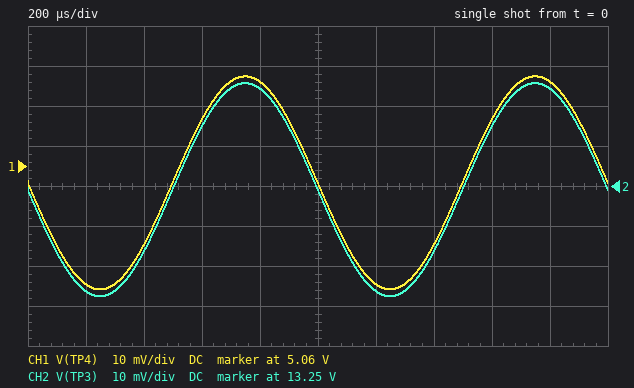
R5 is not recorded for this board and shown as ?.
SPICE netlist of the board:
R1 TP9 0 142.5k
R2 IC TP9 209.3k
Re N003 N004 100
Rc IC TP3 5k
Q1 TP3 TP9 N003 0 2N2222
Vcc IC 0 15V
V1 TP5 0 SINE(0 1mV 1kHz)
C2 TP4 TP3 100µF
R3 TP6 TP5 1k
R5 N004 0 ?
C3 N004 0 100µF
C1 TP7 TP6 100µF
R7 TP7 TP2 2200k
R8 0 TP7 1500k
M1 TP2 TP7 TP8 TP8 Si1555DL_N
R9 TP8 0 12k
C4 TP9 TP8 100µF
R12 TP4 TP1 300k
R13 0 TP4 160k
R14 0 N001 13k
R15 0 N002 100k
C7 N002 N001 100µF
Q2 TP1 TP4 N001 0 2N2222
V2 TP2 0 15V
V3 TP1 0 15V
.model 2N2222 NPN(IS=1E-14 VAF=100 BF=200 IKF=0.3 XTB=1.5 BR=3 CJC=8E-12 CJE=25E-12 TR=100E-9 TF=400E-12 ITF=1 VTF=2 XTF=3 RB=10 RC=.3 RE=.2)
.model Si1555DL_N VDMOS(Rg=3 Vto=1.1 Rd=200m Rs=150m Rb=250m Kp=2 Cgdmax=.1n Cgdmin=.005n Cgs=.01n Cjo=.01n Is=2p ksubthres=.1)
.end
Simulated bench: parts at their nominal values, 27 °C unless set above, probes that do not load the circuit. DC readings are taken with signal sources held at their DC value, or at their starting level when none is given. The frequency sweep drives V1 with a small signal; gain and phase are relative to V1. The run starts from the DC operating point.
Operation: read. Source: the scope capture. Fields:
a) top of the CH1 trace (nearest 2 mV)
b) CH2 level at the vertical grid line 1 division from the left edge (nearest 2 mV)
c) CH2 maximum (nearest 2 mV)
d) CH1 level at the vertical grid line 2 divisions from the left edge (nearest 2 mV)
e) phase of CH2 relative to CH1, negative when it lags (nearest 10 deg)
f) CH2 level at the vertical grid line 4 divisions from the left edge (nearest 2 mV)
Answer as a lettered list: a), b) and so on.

a) 5.082 V
b) 13.224 V
c) 13.276 V
d) 5.040 V
e) 0 deg
f) 13.274 V
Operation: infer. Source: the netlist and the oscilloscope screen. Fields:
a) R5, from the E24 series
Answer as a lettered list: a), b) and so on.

a) 15 kΩ
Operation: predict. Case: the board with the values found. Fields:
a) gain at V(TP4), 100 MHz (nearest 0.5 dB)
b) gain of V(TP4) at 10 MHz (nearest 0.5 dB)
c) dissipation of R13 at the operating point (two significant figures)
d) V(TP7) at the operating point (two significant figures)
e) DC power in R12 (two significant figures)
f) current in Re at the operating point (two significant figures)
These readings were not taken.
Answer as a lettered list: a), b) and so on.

a) -23.0 dB
b) 16.5 dB
c) 160 µW
d) 6.1 V
e) 330 µW
f) 350 µA
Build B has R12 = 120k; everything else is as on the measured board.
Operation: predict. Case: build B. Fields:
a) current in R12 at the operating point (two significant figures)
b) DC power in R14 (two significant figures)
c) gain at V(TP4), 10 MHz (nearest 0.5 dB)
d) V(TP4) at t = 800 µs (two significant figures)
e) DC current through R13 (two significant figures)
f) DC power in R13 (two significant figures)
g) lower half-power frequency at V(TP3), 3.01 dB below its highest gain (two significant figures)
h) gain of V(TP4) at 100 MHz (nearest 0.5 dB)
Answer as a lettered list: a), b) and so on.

a) 55 µA
b) 4.6 mW
c) 16.0 dB
d) 8.4 V
e) 52 µA
f) 440 µW
g) 9.2 Hz
h) -23.5 dB
